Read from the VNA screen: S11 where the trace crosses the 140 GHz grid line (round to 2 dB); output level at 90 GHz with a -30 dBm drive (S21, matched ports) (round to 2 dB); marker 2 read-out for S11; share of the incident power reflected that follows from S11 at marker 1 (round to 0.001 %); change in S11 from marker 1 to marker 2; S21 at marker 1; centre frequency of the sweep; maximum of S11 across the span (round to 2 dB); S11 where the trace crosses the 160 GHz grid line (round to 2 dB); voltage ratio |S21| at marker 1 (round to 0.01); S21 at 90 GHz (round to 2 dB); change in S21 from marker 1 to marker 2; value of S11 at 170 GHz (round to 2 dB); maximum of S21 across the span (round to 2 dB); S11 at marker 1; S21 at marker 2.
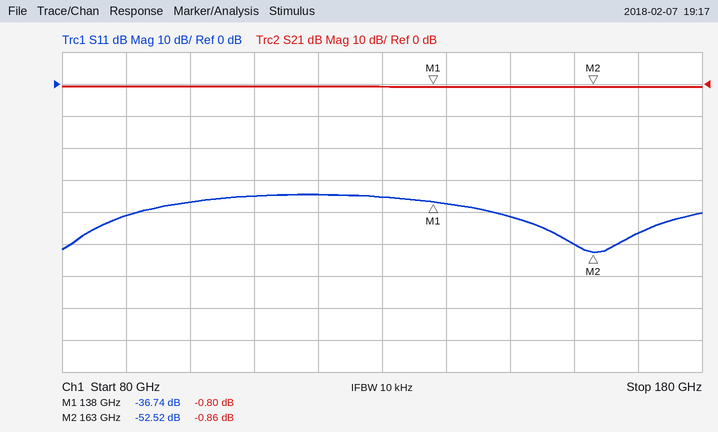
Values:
-38 dB
-30 dBm
-52.52 dB
0.021 %
-15.78 dB
-0.80 dB
130 GHz
-34 dB
-50 dB
0.91
0 dB
-0.06 dB
-46 dB
0 dB
-36.74 dB
-0.86 dB
